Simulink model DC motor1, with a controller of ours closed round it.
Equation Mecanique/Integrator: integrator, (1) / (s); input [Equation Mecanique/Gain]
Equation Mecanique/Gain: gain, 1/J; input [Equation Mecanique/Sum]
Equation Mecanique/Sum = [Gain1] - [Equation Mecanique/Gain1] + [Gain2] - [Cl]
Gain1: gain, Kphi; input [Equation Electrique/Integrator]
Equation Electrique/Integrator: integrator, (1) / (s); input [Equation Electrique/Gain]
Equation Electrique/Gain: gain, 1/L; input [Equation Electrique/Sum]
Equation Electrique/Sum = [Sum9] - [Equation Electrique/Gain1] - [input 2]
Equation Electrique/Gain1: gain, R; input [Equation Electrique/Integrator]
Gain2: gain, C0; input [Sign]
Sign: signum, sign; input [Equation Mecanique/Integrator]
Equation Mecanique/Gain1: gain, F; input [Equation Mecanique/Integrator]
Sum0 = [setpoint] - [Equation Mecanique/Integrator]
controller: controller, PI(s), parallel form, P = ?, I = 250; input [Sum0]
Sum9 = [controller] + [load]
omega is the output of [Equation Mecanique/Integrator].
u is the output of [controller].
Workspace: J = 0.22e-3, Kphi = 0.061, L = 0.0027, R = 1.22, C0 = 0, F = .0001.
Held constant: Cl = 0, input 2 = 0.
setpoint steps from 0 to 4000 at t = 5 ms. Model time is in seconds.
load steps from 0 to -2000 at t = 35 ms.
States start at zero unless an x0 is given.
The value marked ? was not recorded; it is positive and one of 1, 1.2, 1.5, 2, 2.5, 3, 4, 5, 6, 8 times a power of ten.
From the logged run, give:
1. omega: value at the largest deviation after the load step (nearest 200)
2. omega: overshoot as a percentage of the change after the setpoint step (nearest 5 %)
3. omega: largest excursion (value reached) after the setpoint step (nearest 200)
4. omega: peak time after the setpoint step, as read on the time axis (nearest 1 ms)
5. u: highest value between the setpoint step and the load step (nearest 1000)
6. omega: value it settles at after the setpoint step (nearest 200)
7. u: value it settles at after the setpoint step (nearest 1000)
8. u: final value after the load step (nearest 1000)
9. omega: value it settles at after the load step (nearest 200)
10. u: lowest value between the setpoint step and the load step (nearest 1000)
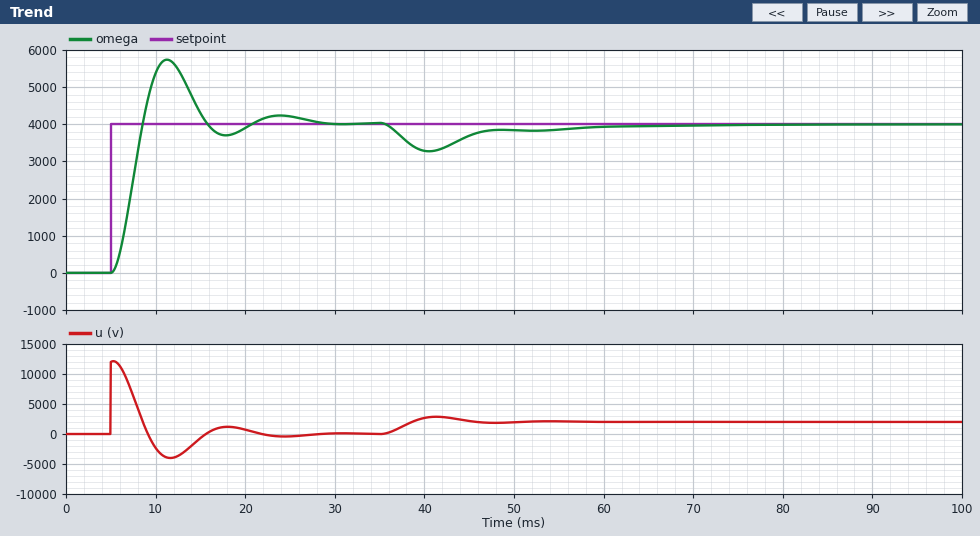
3200
45 %
5800
11 ms
12000
4000
0
2000
4000
-4000
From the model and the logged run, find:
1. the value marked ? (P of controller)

3
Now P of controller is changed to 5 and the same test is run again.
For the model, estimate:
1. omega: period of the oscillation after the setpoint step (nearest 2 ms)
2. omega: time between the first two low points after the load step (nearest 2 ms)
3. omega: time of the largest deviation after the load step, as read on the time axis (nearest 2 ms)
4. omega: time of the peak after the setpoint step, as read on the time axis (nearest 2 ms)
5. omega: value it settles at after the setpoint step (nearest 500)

10 ms
8 ms
40 ms
10 ms
4000
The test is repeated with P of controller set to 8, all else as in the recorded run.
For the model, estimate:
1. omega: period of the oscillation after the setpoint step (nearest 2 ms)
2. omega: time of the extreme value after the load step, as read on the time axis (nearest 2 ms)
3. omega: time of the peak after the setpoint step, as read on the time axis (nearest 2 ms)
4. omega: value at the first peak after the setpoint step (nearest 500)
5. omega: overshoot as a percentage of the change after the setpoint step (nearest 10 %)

8 ms
38 ms
8 ms
6000
50 %
